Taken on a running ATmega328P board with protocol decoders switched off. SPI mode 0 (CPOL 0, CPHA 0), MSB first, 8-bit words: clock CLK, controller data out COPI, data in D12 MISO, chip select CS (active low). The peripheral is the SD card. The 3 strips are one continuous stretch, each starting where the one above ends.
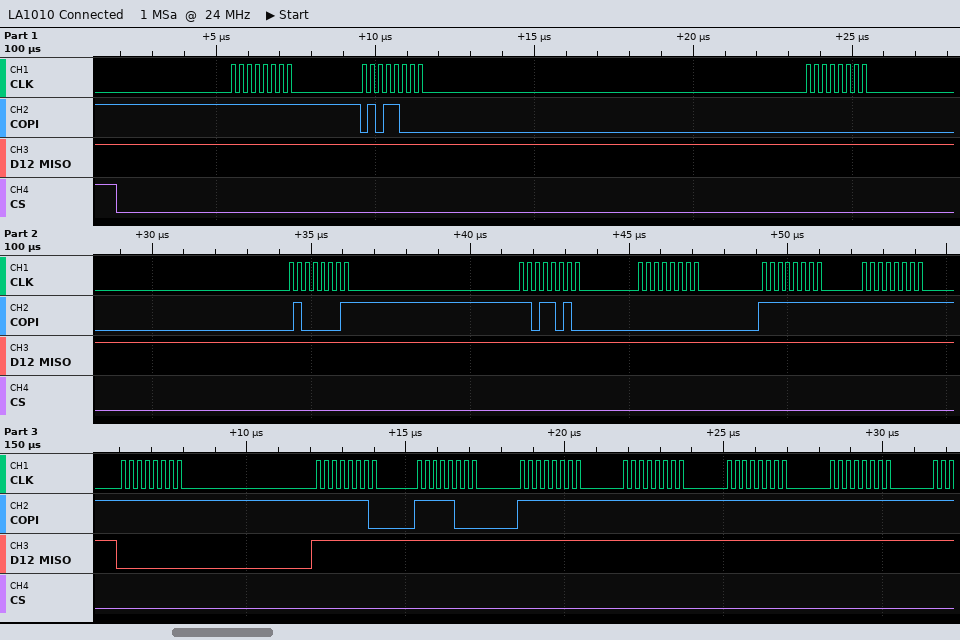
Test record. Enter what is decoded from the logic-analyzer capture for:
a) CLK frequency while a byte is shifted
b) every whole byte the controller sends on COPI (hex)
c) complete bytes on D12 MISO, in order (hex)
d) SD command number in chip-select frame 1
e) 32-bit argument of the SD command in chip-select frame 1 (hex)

4 MHz
FF 58 00 41 DA 00 FF FF FF FE F8 FF FF FF FF
FF FF FF FF FF FF FF FF 00 FF FF FF FF FF FF
CMD24
0x0041DA00
